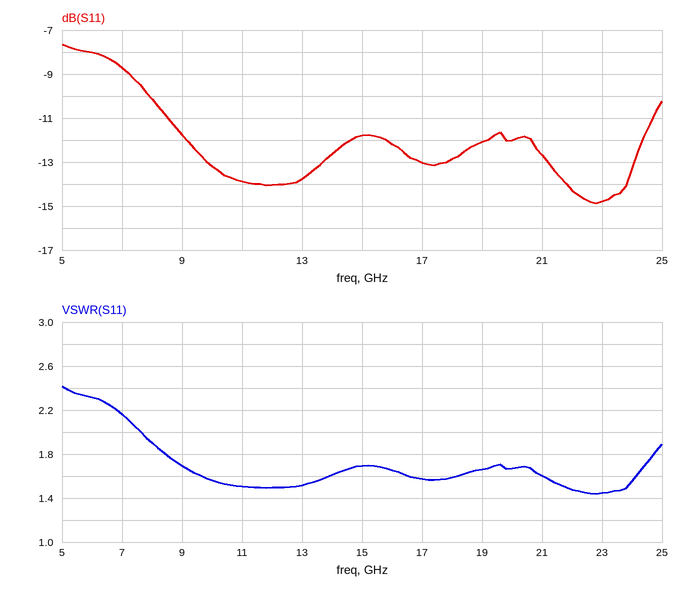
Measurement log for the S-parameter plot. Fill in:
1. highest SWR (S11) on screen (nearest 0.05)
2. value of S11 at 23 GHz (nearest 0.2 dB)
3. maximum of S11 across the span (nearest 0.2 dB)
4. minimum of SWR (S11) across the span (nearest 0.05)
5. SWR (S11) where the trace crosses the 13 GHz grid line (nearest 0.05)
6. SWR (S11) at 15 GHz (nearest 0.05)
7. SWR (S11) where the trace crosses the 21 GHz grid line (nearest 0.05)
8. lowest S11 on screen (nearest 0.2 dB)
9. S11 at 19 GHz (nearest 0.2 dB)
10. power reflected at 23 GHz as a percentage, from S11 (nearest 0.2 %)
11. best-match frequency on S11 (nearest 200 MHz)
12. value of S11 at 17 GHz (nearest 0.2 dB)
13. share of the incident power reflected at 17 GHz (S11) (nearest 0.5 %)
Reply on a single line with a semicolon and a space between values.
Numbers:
2.40; -14.8 dB; -7.6 dB; 1.45; 1.50; 1.70; 1.60; -14.8 dB; -12.0 dB; 3.4 %; 22.8 GHz; -13.0 dB; 5.0 %
